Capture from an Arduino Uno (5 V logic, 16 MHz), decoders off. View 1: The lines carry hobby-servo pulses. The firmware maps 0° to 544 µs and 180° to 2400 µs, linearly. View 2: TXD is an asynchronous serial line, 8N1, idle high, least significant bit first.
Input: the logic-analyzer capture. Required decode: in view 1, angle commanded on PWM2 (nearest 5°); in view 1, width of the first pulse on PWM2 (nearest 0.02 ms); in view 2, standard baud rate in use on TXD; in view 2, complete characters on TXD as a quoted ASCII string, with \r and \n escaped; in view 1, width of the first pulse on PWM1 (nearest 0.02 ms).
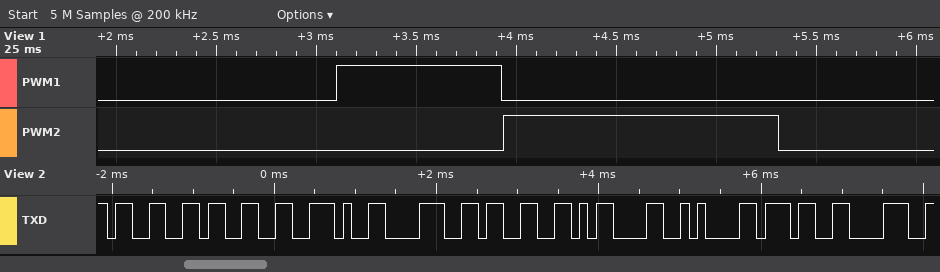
80°
1.38 ms
9600 baud
"33.83\r\n78"
0.82 ms
